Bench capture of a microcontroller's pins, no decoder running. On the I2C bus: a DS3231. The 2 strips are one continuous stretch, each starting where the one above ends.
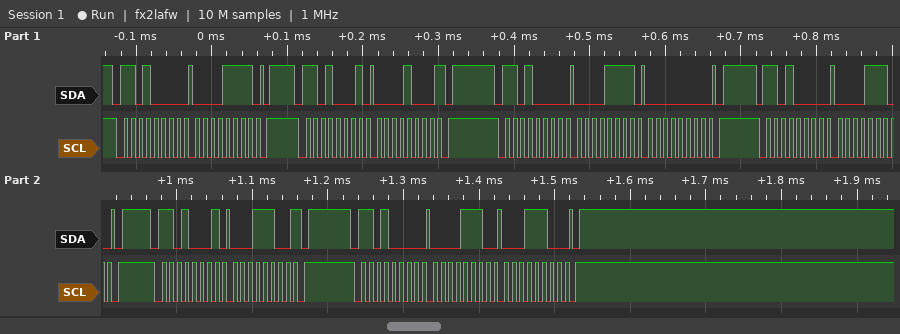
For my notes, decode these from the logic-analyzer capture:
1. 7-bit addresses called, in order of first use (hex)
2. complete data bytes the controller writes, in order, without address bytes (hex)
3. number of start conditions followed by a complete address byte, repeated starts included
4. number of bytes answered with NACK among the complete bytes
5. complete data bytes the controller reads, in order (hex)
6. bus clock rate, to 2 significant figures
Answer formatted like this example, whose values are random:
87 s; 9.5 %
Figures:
0x68; 0F 0F 00 0E 0E 1C; 6; 2; 08 1C; 100 kHz
